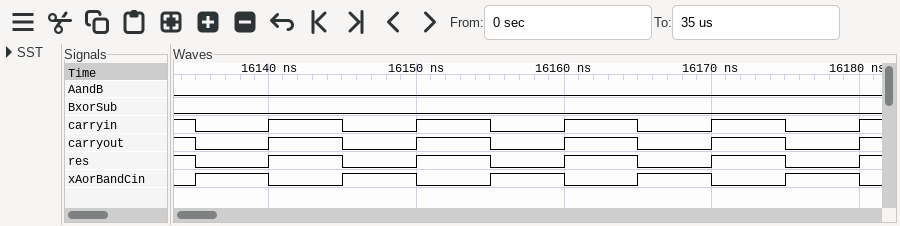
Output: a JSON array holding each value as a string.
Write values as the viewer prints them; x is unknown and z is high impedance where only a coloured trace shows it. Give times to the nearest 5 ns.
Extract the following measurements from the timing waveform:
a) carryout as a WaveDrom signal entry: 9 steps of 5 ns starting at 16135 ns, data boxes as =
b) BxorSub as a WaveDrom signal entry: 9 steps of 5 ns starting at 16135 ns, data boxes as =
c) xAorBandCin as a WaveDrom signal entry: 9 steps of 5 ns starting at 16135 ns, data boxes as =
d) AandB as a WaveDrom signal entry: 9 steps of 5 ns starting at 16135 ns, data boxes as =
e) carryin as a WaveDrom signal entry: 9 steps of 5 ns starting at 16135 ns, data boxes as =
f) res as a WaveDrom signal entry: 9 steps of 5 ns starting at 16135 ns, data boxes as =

["{name: 'carryout', wave: '010101010'}", "{name: 'BxorSub', wave: '0........'}", "{name: 'xAorBandCin', wave: '101010101'}", "{name: 'AandB', wave: '0........'}", "{name: 'carryin', wave: '010101010'}", "{name: 'res', wave: '010101010'}"]
